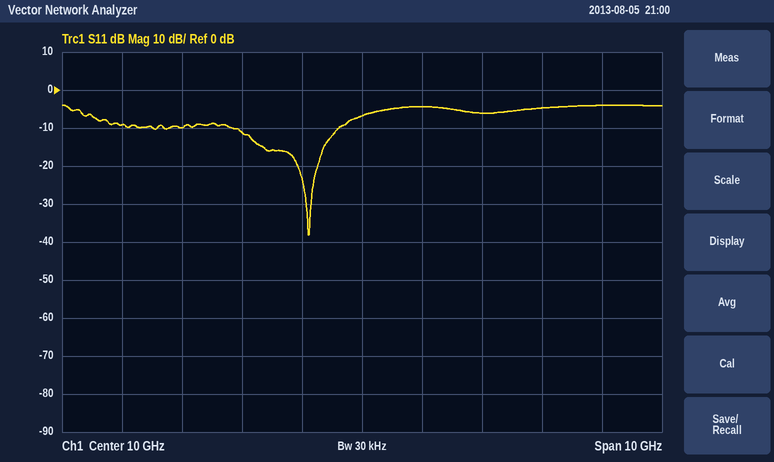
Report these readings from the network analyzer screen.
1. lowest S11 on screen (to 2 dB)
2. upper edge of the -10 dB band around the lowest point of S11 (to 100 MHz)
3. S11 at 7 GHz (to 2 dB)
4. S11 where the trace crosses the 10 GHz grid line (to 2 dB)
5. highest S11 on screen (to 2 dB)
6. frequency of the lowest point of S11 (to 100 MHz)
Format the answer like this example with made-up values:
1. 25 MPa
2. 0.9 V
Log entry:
1. -38 dB
2. 9.6 GHz
3. -10 dB
4. -6 dB
5. -4 dB
6. 9.1 GHz
